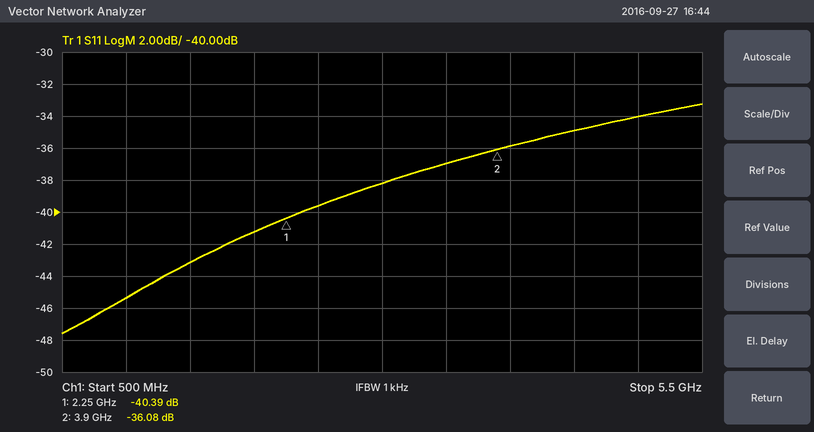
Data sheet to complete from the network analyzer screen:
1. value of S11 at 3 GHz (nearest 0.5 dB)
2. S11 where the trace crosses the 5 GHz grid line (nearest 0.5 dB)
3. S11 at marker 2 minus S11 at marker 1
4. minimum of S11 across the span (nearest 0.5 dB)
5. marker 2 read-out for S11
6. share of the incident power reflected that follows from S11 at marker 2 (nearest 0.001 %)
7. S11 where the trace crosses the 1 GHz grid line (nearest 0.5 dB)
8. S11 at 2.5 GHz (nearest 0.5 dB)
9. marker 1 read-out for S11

-38.0 dB
-34.0 dB
4.31 dB
-47.5 dB
-36.08 dB
0.025 %
-45.5 dB
-39.5 dB
-40.39 dB
